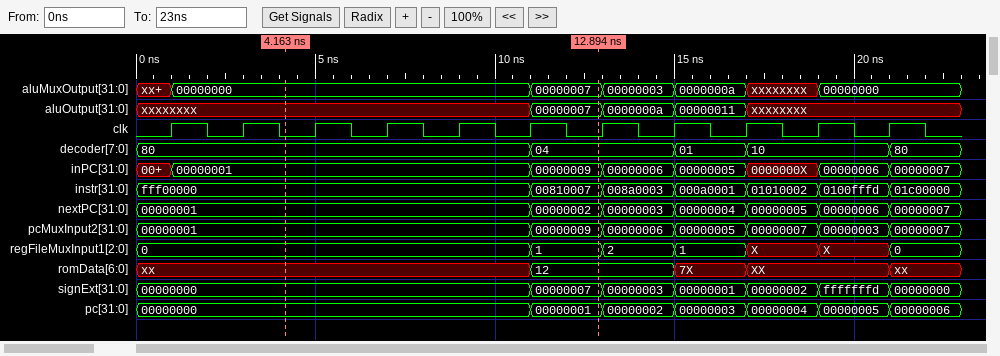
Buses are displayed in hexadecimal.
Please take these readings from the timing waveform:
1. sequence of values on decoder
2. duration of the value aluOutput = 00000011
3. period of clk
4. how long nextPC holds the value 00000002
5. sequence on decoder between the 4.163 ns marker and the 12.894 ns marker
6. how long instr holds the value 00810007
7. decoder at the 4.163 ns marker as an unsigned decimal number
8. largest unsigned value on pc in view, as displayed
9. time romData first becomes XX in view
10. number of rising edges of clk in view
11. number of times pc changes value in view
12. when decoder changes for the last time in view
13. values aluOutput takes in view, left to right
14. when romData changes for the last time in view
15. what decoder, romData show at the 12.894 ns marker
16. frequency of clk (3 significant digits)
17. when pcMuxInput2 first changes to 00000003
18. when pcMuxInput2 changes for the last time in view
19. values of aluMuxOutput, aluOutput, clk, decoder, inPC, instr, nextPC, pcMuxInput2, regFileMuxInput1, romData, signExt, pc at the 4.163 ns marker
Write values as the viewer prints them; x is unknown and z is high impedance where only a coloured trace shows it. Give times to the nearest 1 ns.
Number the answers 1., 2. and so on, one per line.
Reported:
1. 80, 04, 01, 10, 80
2. 2 ns
3. 2 ns
4. 2 ns
5. 80, 04
6. 2 ns
7. 128
8. 00000006
9. 17 ns
10. 11
11. 6
12. 21 ns
13. xxxxxxxx, 00000007, 0000000a, 00000011, xxxxxxxx
14. 21 ns
15. decoder=04, romData=12
16. 500 MHz
17. 19 ns
18. 21 ns
19. aluMuxOutput=00000000, aluOutput=xxxxxxxx, clk=0, decoder=80, inPC=00000001, instr=fff00000, nextPC=00000001, pcMuxInput2=00000001, regFileMuxInput1=0, romData=xx, signExt=00000000, pc=00000000
